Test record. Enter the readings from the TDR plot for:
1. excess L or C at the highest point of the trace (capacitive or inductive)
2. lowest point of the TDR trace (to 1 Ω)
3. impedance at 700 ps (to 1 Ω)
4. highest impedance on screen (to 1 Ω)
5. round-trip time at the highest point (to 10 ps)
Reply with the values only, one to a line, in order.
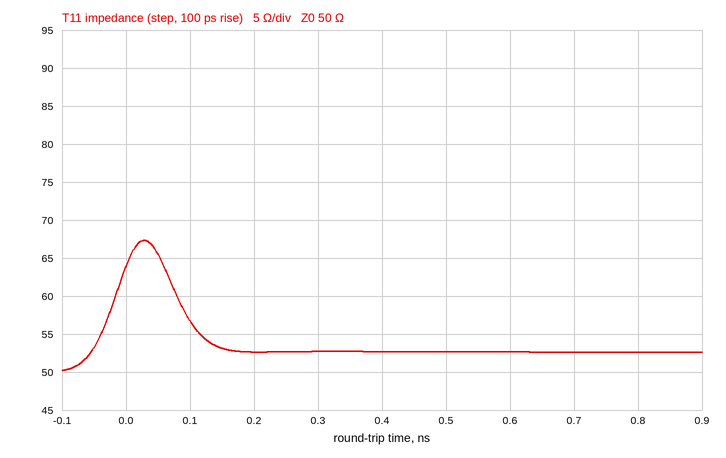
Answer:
inductive
50 Ω
53 Ω
67 Ω
30 ps
